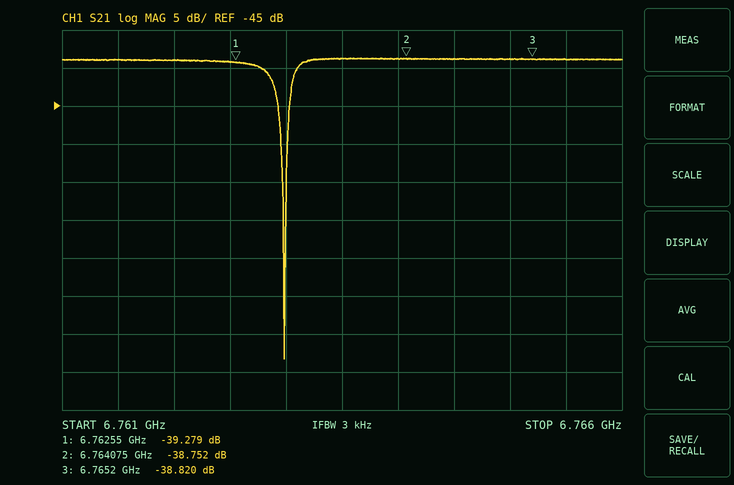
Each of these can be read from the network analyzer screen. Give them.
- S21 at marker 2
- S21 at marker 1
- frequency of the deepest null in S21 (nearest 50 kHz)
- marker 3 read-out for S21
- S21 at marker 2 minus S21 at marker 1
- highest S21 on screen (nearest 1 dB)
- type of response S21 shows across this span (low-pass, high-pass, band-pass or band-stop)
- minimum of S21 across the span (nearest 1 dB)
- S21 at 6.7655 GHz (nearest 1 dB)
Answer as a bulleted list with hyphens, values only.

- -38.752 dB
- -39.279 dB
- 6.76300 GHz
- -38.820 dB
- 0.527 dB
- -39 dB
- band-stop
- -78 dB
- -39 dB
